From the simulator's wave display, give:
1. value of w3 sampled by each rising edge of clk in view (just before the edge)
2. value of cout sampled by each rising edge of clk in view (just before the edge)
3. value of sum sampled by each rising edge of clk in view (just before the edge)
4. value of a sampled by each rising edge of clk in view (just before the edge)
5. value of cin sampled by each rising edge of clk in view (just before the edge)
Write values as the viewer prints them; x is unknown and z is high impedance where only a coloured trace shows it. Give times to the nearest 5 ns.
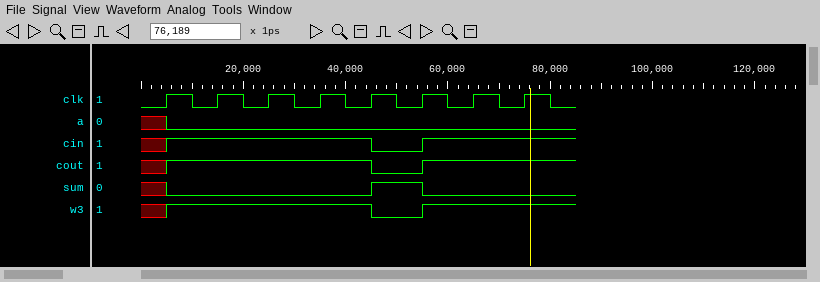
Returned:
x 1 1 1 1 0 1 1
x 1 1 1 1 0 1 1
x 0 0 0 0 1 0 0
x 0 0 0 0 0 0 0
x 1 1 1 1 0 1 1
